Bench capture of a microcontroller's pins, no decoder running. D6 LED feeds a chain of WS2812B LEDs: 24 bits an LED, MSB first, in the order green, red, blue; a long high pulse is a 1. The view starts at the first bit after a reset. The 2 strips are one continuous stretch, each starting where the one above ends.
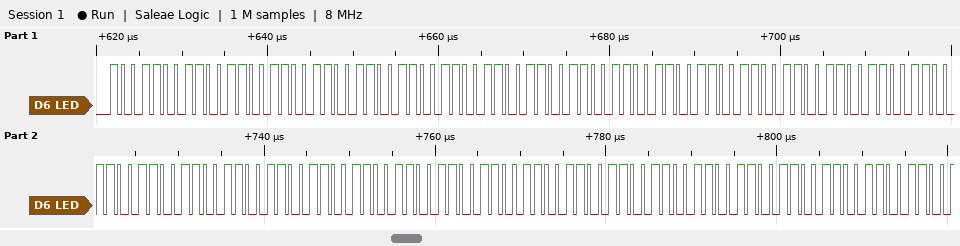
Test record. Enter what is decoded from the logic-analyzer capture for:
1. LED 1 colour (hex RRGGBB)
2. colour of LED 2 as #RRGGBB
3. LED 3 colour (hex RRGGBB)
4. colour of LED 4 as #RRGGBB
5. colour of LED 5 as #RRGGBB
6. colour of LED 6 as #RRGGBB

#999999
#999999
#999999
#999999
#999999
#999999
